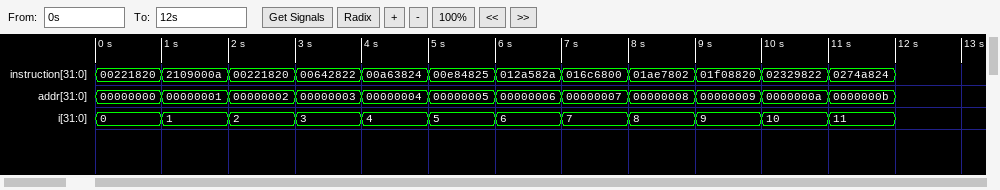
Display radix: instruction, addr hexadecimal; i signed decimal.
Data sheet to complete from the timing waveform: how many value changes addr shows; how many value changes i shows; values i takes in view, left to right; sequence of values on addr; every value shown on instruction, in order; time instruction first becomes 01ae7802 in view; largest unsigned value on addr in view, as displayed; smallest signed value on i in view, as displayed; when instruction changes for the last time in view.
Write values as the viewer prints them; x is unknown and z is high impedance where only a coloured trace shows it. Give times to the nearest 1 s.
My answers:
11
11
0, 1, 2, 3, 4, 5, 6, 7, 8, 9, 10, 11
00000000, 00000001, 00000002, 00000003, 00000004, 00000005, 00000006, 00000007, 00000008, 00000009, 0000000a, 0000000b
00221820, 2109000a, 00221820, 00642822, 00a63824, 00e84825, 012a582a, 016c6800, 01ae7802, 01f08820, 02329822, 0274a824
8 s
0000000b
0
11 s
